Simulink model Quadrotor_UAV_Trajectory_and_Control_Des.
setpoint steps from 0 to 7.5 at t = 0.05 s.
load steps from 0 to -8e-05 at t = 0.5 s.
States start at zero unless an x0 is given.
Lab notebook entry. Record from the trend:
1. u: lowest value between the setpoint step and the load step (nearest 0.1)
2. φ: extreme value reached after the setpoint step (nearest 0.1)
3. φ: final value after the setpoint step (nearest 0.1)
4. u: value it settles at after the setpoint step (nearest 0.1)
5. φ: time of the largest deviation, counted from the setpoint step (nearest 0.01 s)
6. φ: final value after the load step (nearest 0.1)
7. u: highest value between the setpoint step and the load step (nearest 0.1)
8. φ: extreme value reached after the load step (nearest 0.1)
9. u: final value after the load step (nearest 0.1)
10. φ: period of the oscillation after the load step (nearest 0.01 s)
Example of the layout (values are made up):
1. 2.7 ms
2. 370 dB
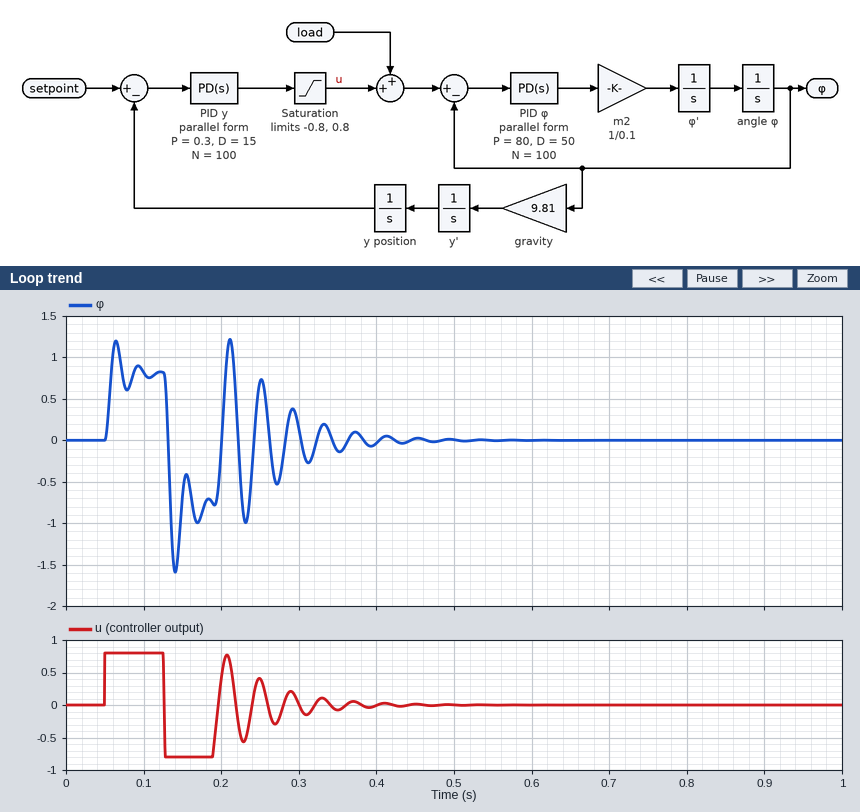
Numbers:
1. -0.8
2. -1.6
3. 0.0
4. 0.0
5. 0.09 s
6. 0.0
7. 0.8
8. 0.0
9. 0.0
10. 0.04 s
